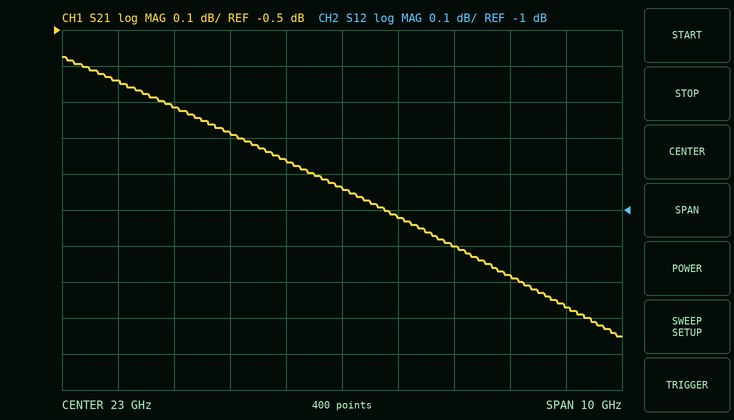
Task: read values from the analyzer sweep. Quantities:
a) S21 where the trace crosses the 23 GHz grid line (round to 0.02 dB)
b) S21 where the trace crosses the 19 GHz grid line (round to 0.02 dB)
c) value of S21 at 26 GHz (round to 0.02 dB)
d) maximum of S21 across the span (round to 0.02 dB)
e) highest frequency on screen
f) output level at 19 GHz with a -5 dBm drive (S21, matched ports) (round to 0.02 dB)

-0.94 dB
-0.64 dB
-1.18 dB
-0.58 dB
28 GHz
-5.64 dBm
